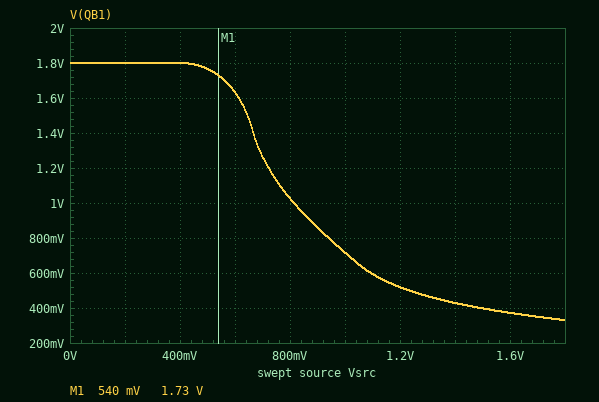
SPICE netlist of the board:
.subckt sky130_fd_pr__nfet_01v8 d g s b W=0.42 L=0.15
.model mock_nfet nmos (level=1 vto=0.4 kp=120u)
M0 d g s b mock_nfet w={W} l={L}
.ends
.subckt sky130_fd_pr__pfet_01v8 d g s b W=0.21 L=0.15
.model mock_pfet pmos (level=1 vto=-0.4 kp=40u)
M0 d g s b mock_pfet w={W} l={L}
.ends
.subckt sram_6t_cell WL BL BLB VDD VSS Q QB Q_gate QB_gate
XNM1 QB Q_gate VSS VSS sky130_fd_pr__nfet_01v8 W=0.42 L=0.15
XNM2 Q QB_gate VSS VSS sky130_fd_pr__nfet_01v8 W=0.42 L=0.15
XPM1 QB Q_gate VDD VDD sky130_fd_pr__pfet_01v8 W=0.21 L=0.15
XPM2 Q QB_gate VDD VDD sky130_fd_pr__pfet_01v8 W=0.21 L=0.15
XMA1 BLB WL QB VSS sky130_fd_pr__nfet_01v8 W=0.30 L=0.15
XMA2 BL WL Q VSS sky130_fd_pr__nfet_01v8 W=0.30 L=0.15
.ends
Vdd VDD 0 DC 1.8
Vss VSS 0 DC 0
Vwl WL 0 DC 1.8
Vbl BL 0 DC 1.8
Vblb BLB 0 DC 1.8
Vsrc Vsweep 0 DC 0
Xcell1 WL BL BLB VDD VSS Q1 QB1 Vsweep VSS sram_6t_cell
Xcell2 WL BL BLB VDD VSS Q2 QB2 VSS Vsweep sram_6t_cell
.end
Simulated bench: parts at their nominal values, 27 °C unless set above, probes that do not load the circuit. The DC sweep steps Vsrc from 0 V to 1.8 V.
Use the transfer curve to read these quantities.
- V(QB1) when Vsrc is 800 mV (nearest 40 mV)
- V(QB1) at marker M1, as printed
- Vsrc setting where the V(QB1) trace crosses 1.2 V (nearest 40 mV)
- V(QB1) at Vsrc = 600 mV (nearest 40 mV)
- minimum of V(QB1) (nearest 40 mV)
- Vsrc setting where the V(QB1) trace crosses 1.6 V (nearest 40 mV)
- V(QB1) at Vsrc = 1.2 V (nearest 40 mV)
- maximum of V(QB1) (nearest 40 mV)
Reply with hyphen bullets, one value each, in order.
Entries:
- 1.04 V
- 1.73 V
- 720 mV
- 1.64 V
- 320 mV
- 600 mV
- 520 mV
- 1.80 V
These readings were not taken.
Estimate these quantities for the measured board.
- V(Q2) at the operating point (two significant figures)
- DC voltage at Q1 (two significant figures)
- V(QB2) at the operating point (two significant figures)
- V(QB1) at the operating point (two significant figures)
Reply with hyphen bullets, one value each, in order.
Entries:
- 1.8 V
- 1.8 V
- 1.8 V
- 1.8 V
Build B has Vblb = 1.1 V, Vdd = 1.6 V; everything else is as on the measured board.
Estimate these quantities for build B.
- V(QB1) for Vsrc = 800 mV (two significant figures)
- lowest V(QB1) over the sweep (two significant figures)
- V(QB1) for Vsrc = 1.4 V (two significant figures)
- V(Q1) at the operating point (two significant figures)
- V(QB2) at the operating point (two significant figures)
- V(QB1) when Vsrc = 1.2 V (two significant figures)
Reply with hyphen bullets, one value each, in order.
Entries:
- 870 mV
- 310 mV
- 400 mV
- 1.6 V
- 1.4 V
- 480 mV
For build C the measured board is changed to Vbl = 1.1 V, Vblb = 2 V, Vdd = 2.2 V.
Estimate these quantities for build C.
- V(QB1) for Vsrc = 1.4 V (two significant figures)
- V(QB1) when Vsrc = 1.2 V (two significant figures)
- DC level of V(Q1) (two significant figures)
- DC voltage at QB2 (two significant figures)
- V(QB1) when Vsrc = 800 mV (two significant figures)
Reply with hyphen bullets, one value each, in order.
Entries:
- 440 mV
- 550 mV
- 2.1 V
- 2.2 V
- 1.4 V
